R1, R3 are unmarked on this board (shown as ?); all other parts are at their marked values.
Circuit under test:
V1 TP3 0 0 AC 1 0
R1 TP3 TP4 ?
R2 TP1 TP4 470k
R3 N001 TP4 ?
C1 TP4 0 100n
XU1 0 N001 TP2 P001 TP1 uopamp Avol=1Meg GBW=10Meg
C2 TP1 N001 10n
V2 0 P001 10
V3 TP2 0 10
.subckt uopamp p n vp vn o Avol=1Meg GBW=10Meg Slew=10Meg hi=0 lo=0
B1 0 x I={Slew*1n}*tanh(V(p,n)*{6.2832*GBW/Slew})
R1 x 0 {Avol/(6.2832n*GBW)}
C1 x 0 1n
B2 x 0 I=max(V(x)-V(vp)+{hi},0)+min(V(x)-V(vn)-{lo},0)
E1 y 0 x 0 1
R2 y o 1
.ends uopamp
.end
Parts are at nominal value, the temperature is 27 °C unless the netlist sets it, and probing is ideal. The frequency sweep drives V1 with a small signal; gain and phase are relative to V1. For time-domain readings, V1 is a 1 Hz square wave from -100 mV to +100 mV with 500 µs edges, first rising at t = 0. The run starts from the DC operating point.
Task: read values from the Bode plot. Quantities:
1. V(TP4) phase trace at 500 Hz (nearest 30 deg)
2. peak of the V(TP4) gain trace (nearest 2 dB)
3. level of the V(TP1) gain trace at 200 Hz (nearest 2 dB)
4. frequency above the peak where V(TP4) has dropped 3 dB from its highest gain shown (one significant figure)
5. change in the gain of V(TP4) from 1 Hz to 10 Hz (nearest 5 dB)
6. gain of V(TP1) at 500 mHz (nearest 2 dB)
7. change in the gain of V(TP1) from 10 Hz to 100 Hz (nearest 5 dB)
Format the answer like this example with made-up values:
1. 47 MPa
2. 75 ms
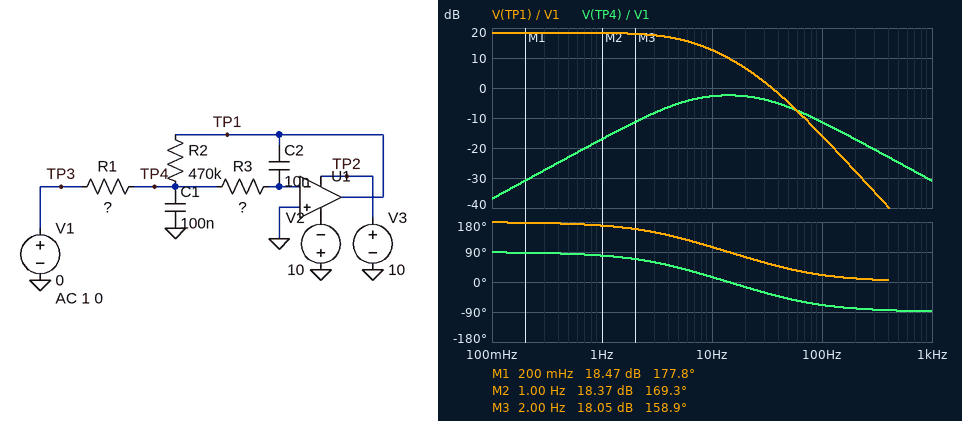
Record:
1. -90 deg
2. -2 dB
3. -28 dB
4. 40 Hz
5. 15 dB
6. 18 dB
7. -30 dB
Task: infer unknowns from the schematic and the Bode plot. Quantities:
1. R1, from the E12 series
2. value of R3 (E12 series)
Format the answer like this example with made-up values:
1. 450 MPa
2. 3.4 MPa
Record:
1. 56 kΩ
2. 270 kΩ
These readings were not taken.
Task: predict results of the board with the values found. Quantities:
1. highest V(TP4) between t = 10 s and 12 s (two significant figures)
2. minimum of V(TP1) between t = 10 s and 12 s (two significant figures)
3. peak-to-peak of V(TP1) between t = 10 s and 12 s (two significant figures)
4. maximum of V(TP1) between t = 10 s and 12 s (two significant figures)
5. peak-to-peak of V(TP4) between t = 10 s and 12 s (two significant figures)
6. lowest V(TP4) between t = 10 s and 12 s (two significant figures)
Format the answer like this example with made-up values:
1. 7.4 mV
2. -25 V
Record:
1. 120 mV
2. -840 mV
3. 1.7 V
4. 840 mV
5. 240 mV
6. -120 mV
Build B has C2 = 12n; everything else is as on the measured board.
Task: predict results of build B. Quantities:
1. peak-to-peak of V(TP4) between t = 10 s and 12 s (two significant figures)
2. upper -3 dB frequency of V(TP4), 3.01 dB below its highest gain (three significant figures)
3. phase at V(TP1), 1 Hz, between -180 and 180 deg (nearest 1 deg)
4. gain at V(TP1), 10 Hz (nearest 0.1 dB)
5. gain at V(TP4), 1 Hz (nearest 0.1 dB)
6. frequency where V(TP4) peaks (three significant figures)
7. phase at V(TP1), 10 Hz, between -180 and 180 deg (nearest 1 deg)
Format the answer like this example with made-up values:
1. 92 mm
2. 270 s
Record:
1. 250 mV
2. 41.7 Hz
3. 167 deg
4. 11.2 dB
5. -15.5 dB
6. 12.9 Hz
7. 100 deg
